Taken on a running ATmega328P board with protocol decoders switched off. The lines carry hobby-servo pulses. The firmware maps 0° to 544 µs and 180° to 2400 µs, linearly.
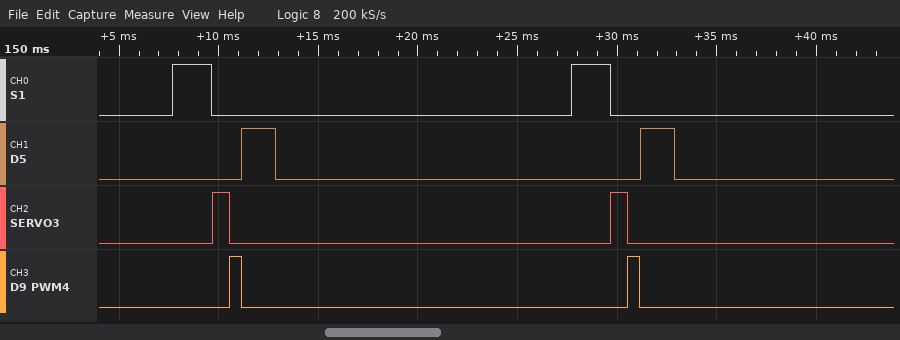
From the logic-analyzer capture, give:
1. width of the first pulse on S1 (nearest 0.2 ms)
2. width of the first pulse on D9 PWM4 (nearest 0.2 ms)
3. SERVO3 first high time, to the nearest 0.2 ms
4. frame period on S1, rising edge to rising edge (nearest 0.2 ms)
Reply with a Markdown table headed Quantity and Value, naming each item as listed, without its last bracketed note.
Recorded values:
| Quantity | Value |
|---|---|
| width of the first pulse on S1 | 2.0 ms |
| width of the first pulse on D9 PWM4 | 0.6 ms |
| SERVO3 first high time, to the nearest 0.2 ms | 0.8 ms |
| frame period on S1, rising edge to rising edge | 20.0 ms |
